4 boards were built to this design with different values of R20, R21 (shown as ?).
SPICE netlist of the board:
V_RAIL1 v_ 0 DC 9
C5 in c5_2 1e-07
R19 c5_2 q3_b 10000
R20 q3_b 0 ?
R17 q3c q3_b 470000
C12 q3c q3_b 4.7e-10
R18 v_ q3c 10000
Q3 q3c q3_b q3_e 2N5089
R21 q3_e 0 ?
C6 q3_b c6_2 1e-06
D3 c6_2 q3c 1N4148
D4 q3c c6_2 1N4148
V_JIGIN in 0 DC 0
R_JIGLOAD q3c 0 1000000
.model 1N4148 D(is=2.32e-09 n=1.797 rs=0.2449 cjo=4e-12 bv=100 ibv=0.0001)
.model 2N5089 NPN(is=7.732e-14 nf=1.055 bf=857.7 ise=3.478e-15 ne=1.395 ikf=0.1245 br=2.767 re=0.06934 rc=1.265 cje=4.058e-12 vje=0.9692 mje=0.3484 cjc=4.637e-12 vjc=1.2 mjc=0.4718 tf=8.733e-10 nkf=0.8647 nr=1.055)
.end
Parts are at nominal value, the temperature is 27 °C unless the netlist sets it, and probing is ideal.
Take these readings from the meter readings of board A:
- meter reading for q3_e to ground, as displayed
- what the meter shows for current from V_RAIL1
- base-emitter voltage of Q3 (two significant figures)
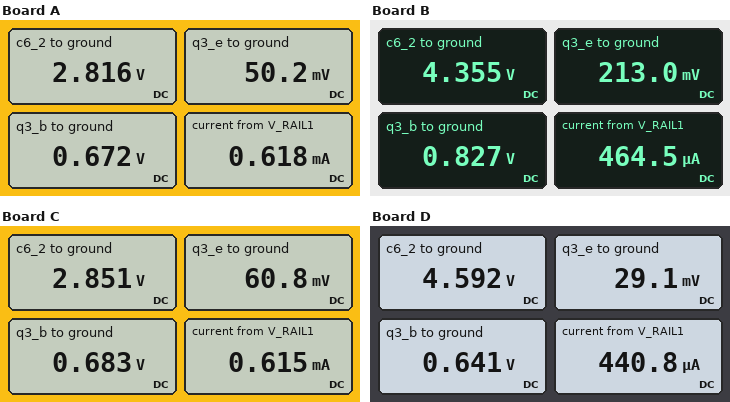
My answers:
50.2 mV
0.618 mA
620 mV
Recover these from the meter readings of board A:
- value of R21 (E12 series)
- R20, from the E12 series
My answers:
82 Ω
180 kΩ
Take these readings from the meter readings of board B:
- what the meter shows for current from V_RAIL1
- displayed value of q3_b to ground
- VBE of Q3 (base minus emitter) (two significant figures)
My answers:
464.5 µA
0.827 V
610 mV
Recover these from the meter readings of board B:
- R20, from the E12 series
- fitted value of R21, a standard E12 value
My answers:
120 kΩ
470 Ω
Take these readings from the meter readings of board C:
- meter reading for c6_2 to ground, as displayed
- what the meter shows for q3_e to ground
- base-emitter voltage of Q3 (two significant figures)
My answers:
2.851 V
60.8 mV
620 mV
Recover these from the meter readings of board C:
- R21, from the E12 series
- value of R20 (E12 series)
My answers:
100 Ω
180 kΩ
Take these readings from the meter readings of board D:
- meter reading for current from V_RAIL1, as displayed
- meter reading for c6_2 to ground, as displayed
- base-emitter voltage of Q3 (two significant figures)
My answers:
440.8 µA
4.592 V
610 mV
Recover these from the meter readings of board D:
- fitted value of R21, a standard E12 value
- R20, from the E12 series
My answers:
68 Ω
82 kΩ
